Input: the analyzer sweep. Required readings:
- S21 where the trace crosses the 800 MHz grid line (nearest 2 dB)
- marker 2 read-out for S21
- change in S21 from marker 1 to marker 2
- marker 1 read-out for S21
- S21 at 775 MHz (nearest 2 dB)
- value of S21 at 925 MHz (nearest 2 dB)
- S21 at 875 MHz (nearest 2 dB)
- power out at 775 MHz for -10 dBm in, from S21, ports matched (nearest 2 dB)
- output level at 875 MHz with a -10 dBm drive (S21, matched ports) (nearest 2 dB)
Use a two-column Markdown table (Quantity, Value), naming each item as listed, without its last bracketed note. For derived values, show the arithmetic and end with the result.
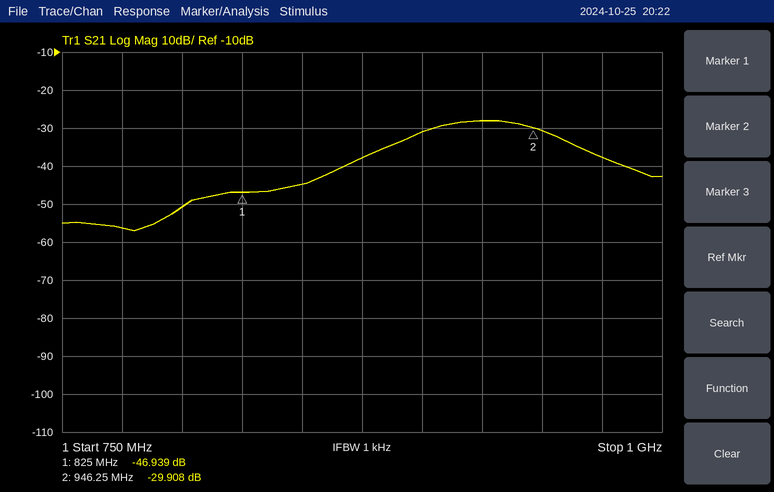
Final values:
| Quantity | Value |
|---|---|
| S21 where the trace crosses the 800 MHz grid line | -50 dB |
| marker 2 read-out for S21 | -29.908 dB |
| change in S21 from marker 1 to marker 2 | -29.908 − (-46.939) = 17.031 dB |
| marker 1 read-out for S21 | -46.939 dB |
| S21 at 775 MHz | -56 dB |
| value of S21 at 925 MHz | -28 dB |
| S21 at 875 MHz | -38 dB |
| power out at 775 MHz for -10 dBm in, from S21, ports matched | -10 dBm + (-56 dB) = -66 dBm |
| output level at 875 MHz with a -10 dBm drive (S21, matched ports) | -10 dBm + (-38 dB) = -48 dBm |
